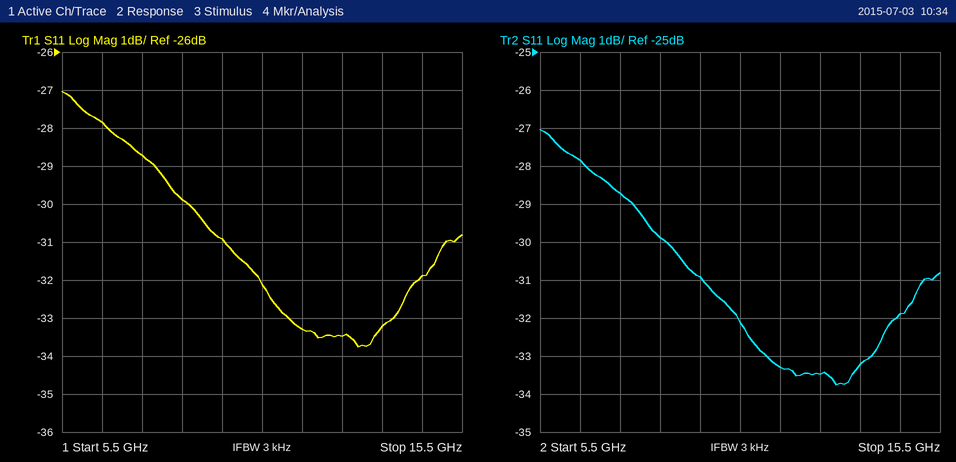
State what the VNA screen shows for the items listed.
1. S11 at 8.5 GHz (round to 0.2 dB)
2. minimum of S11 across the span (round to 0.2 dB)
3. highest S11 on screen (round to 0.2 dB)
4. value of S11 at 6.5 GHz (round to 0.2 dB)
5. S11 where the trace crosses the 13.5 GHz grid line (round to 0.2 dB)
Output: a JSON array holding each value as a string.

["-29.8 dB", "-33.8 dB", "-27.0 dB", "-27.8 dB", "-33.2 dB"]
